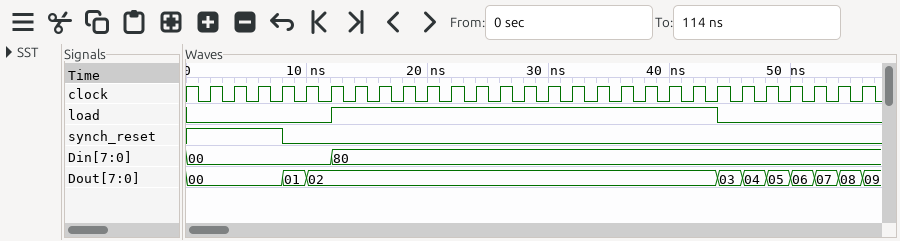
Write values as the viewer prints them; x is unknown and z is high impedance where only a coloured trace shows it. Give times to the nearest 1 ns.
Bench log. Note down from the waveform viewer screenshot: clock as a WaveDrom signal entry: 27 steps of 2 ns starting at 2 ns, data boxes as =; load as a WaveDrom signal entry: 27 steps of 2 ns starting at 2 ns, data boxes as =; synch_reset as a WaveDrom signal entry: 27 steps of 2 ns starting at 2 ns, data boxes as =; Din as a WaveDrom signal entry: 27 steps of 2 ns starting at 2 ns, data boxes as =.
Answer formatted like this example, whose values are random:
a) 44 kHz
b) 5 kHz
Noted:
a) {name: 'clock', wave: 'p..........................'}
b) {name: 'load', wave: '0....1...............0.....'}
c) {name: 'synch_reset', wave: '1..0.......................'}
d) {name: 'Din', wave: '=....=.....................', data: '00 80'}
